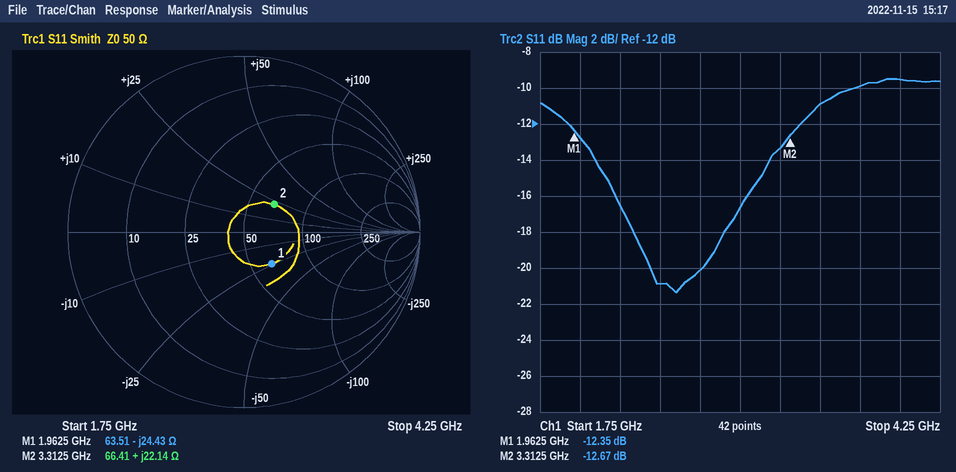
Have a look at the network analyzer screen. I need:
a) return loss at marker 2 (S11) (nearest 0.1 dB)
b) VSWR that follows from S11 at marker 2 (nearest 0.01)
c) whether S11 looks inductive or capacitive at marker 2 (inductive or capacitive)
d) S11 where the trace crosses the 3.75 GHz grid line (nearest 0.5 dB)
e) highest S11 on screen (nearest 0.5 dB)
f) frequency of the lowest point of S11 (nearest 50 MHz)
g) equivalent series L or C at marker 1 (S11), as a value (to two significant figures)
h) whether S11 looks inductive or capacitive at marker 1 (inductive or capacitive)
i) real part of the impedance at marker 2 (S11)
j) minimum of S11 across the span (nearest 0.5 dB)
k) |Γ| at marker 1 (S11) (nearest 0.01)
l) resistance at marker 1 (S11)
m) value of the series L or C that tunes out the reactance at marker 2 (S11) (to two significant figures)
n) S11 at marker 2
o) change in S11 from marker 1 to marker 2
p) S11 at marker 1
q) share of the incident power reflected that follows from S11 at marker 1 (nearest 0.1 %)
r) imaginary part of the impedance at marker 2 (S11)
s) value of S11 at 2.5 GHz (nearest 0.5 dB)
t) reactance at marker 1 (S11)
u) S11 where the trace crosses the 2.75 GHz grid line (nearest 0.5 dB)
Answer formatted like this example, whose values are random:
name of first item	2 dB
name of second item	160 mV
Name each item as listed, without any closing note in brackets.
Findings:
return loss at marker 2 (S11)	12.7 dB
VSWR that follows from S11 at marker 2	1.61
whether S11 looks inductive or capacitive at marker 2	inductive
S11 where the trace crosses the 3.75 GHz grid line	-10.0 dB
highest S11 on screen	-9.5 dB
frequency of the lowest point of S11	2.60 GHz
equivalent series L or C at marker 1 (S11), as a value	3.3 pF
whether S11 looks inductive or capacitive at marker 1	capacitive
real part of the impedance at marker 2	66.41 Ω
minimum of S11 across the span	-21.5 dB
|Γ| at marker 1 (S11)	0.24
resistance at marker 1	63.51 Ω
value of the series L or C that tunes out the reactance at marker 2 (S11)	2.2 pF
S11 at marker 2	-12.67 dB
change in S11 from marker 1 to marker 2	-0.32 dB
S11 at marker 1	-12.35 dB
share of the incident power reflected that follows from S11 at marker 1	5.8 %
imaginary part of the impedance at marker 2	+22.14 Ω
value of S11 at 2.5 GHz	-21.0 dB
reactance at marker 1	-24.43 Ω
S11 where the trace crosses the 2.75 GHz grid line	-20.0 dB
